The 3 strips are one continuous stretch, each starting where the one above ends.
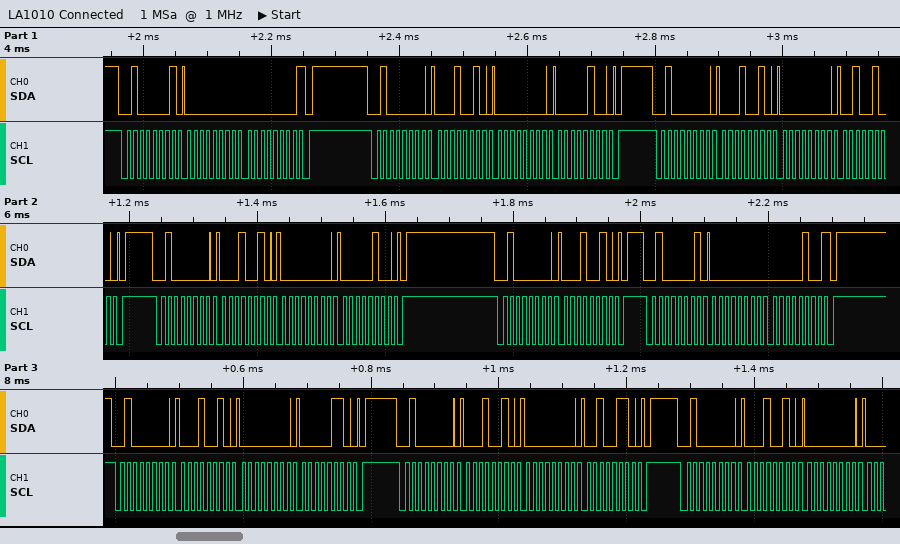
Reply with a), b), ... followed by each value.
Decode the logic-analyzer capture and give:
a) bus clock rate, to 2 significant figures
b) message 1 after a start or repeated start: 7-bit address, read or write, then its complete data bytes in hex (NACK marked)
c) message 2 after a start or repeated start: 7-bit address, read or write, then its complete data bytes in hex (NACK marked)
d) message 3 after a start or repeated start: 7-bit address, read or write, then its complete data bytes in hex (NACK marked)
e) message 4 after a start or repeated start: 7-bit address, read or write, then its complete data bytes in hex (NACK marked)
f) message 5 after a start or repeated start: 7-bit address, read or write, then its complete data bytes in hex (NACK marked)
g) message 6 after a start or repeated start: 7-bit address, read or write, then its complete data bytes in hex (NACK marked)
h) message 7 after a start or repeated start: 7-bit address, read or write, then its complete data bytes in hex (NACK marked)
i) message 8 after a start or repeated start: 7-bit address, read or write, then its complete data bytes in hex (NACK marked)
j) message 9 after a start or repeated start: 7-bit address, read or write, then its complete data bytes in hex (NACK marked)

a) 100 kHz
b) 0x20 read: 00 00 NACK
c) 0x20 write: 12 00 04
d) 0x20 write: 12 00 24
e) 0x20 write: 12 00 04
f) 0x20 write: 12
g) 0x20 read: 00 04 NACK
h) 0x20 write: 12 00 06
i) 0x20 write: 12 00 26
j) 0x20 write: 12 00
